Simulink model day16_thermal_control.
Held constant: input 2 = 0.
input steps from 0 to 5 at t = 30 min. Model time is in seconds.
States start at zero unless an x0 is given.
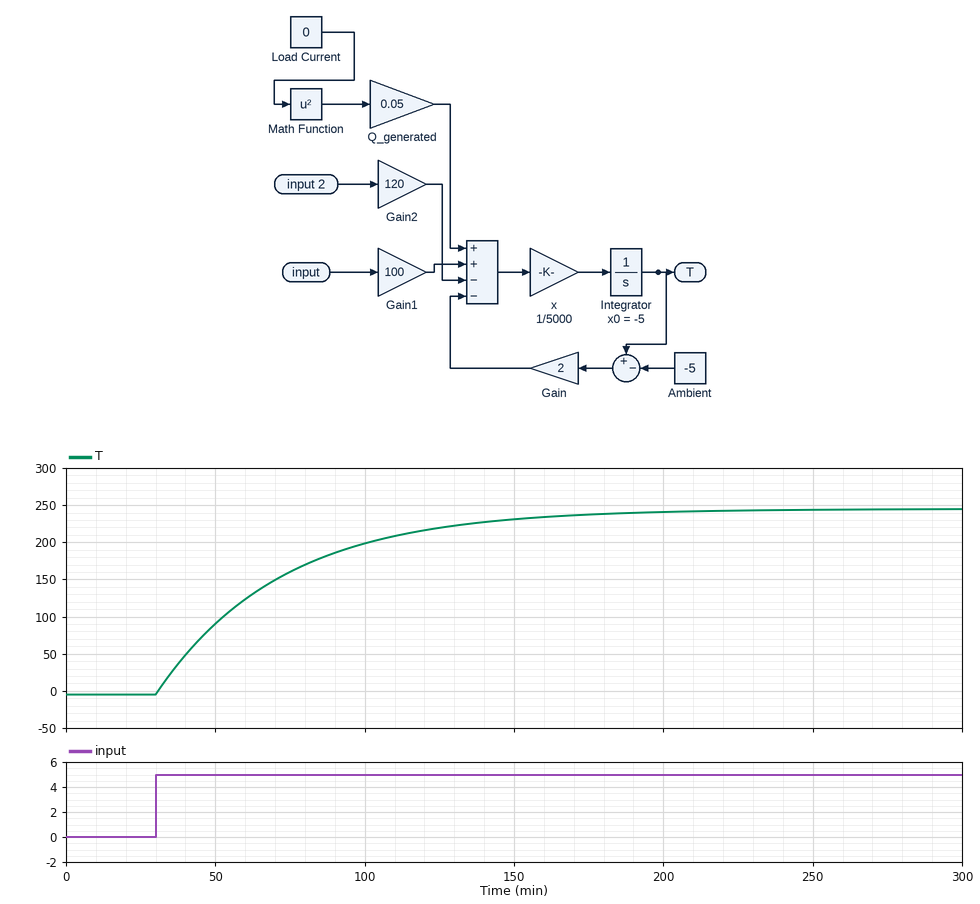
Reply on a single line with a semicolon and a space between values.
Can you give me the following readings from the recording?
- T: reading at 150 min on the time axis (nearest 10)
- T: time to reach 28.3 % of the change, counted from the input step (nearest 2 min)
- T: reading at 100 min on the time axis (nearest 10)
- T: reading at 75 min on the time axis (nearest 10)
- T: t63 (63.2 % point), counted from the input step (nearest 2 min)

230; 14 min; 200; 160; 42 min
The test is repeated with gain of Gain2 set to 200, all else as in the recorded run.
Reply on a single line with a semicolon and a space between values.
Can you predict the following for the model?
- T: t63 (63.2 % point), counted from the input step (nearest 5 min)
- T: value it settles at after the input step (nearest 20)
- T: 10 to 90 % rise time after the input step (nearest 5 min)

40 min; 240; 90 min
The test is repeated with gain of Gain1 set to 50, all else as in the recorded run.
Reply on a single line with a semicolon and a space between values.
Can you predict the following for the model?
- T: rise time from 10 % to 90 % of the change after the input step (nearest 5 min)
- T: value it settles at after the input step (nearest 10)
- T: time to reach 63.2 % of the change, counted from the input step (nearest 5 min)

90 min; 120; 40 min
